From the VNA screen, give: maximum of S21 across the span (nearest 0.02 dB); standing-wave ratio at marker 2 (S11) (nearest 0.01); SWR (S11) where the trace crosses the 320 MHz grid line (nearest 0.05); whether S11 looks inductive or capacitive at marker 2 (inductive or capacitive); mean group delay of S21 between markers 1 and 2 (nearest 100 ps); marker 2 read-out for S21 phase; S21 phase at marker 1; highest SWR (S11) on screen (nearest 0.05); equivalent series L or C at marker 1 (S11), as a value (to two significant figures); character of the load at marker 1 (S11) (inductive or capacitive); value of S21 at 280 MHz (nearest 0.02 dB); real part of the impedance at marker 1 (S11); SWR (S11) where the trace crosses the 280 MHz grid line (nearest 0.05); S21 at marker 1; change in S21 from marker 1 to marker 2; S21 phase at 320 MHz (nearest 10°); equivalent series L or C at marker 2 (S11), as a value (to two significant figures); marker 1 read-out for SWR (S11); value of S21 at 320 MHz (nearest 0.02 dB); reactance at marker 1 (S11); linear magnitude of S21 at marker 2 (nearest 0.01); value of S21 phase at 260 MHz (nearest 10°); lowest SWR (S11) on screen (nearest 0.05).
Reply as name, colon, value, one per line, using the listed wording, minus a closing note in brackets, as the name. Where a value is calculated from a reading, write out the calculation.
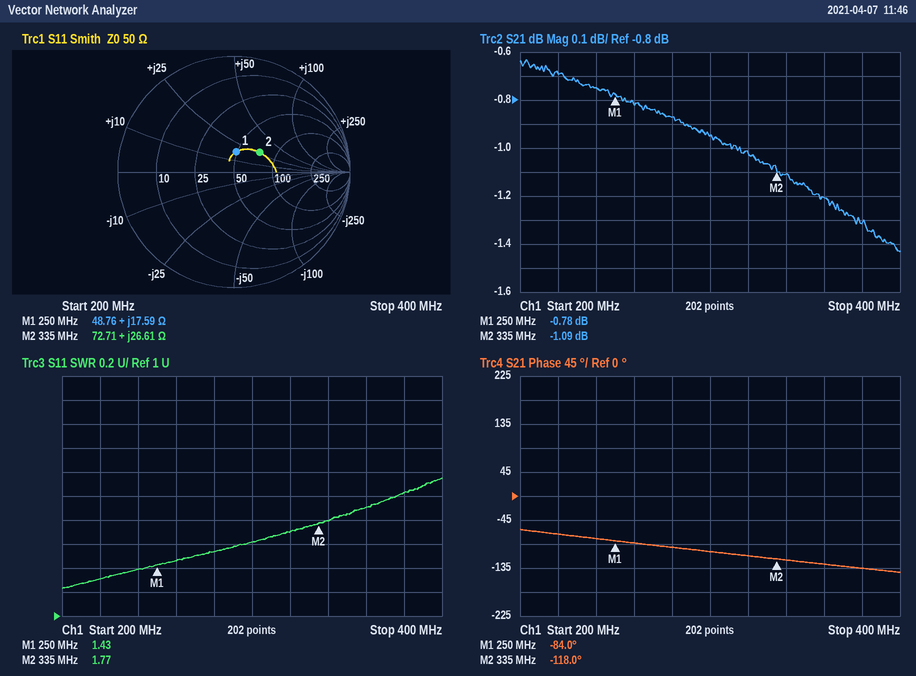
maximum of S21 across the span: -0.64 dB
standing-wave ratio at marker 2 (S11): 1.77
SWR (S11) where the trace crosses the 320 MHz grid line: 1.70
whether S11 looks inductive or capacitive at marker 2: inductive
mean group delay of S21 between markers 1 and 2: −(-118° − (-84°))/(360° × 85 MHz) ≈ 1.1 ns
marker 2 read-out for S21 phase: -118.0°
S21 phase at marker 1: -84.0°
highest SWR (S11) on screen: 2.15
equivalent series L or C at marker 1 (S11), as a value: L = 17.59 Ω/(2π × 250 MHz) ≈ 11 nH
character of the load at marker 1 (S11): inductive
value of S21 at 280 MHz: -0.88 dB
real part of the impedance at marker 1: 48.76 Ω
SWR (S11) where the trace crosses the 280 MHz grid line: 1.55
S21 at marker 1: -0.78 dB
change in S21 from marker 1 to marker 2: -1.09 − (-0.78) = -0.31 dB
S21 phase at 320 MHz: -110°
equivalent series L or C at marker 2 (S11), as a value: L = 26.61 Ω/(2π × 335 MHz) ≈ 13 nH
marker 1 read-out for SWR: 1.43
value of S21 at 320 MHz: -1.02 dB
reactance at marker 1: +17.59 Ω
linear magnitude of S21 at marker 2: 10^(-1.09/20) ≈ 0.88
value of S21 phase at 260 MHz: -90°
lowest SWR (S11) on screen: 1.25
